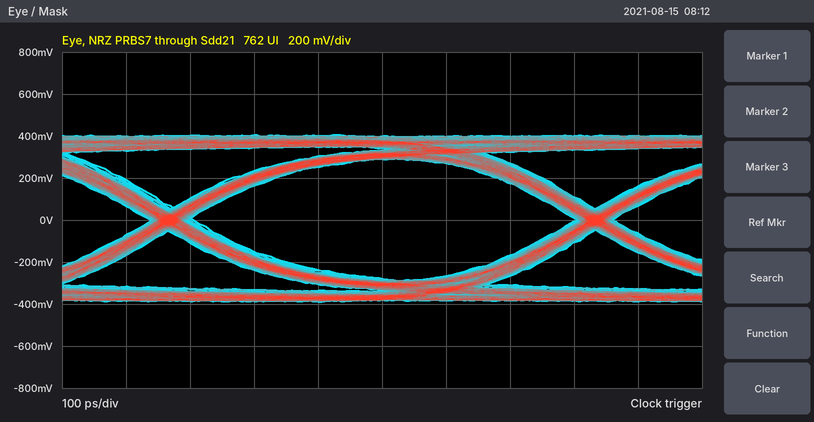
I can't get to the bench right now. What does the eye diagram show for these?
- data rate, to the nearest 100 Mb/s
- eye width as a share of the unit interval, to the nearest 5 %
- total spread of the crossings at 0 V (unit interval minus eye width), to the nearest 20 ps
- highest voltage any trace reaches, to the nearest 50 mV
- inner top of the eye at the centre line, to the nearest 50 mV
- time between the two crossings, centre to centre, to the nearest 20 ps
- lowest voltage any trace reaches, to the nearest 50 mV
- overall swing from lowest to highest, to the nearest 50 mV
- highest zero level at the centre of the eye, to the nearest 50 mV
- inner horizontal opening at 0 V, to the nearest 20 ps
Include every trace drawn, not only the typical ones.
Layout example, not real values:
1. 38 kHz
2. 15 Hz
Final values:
1. 1.5 Gb/s
2. 90 %
3. 60 ps
4. 400 mV
5. 300 mV
6. 660 ps
7. -400 mV
8. 800 mV
9. -300 mV
10. 600 ps
